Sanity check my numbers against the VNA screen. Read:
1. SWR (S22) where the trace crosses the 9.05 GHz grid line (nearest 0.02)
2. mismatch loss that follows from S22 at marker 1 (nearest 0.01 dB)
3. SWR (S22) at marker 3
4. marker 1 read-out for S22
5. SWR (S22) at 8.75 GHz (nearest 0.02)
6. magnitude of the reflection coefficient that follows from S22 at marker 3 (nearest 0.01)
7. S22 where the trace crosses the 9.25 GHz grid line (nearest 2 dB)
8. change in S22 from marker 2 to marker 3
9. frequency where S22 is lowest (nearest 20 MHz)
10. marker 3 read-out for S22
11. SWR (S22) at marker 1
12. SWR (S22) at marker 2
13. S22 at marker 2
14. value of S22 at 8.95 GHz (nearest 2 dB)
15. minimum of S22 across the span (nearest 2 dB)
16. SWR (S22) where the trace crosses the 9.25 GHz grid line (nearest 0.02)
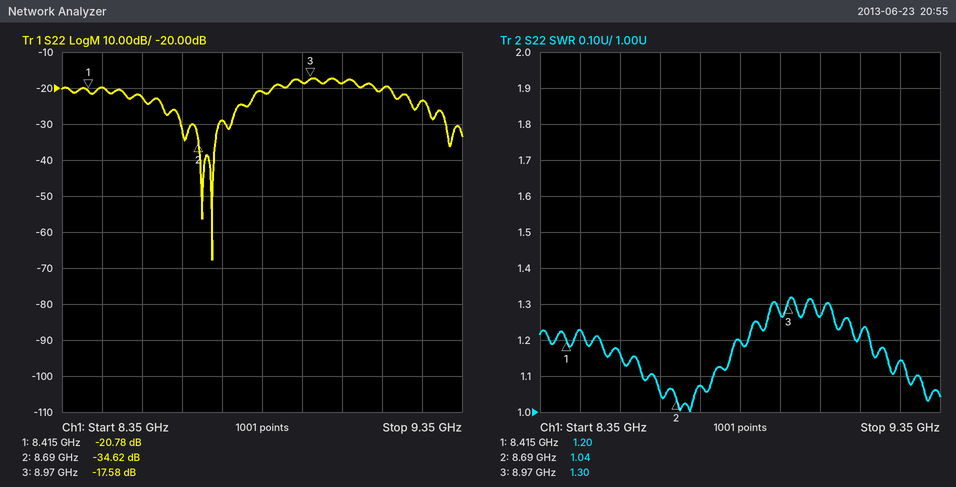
1.26
0.04 dB
1.30
-20.78 dB
1.08
0.13
-24 dB
17.04 dB
8.72 GHz
-17.58 dB
1.20
1.04
-34.62 dB
-18 dB
-68 dB
1.14
